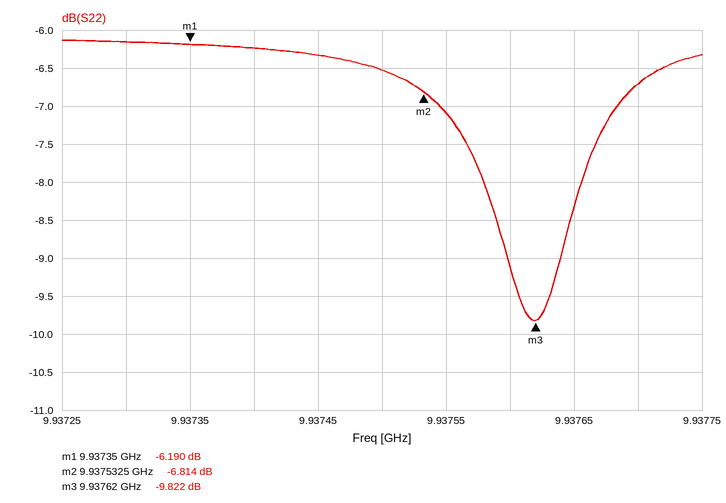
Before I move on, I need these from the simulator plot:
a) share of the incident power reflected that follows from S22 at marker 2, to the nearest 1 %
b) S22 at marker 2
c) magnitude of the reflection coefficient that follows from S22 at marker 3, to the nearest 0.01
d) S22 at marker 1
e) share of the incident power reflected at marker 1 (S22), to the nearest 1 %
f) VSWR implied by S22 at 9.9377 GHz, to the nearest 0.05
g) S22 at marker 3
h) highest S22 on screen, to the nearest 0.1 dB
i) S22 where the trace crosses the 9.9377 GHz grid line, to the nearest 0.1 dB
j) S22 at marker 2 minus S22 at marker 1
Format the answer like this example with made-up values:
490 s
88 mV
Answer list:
21 %
-6.814 dB
0.32
-6.190 dB
24 %
2.70
-9.822 dB
-6.1 dB
-6.7 dB
-0.624 dB
